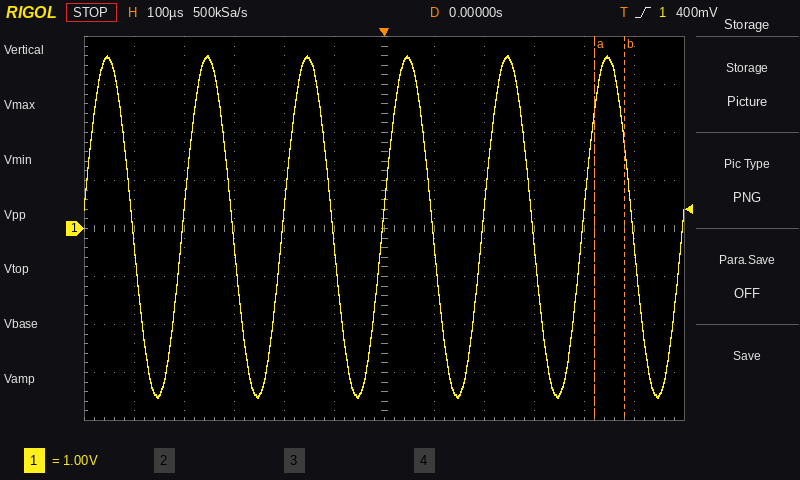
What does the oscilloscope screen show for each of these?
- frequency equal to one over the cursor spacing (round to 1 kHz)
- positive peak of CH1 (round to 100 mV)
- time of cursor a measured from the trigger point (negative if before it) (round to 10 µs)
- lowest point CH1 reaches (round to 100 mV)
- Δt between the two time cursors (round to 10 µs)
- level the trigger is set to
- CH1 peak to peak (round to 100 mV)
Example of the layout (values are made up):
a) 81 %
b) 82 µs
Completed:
a) 17 kHz
b) 3.6 V
c) +420 µs
d) -3.5 V
e) 60 µs
f) 400 mV
g) 7.1 V
